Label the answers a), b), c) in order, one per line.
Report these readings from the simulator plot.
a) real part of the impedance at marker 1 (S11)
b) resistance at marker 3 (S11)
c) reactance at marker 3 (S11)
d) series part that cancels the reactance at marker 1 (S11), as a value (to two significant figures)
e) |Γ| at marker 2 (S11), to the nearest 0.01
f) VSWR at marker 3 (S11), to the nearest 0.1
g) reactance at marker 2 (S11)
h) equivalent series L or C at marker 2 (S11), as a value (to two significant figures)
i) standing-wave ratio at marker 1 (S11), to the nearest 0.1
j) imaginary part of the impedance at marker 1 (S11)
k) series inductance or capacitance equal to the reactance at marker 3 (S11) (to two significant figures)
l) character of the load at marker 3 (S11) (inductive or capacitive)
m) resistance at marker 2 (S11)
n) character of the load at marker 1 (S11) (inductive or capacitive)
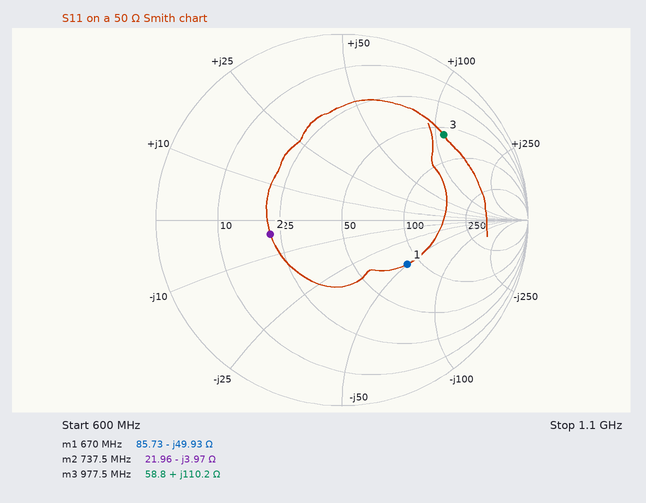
a) 85.73 Ω
b) 58.8 Ω
c) +110.2 Ω
d) 12 nH
e) 0.39
f) 6.0
g) -3.97 Ω
h) 54 pF
i) 2.5
j) -49.93 Ω
k) 18 nH
l) inductive
m) 21.96 Ω
n) capacitive
